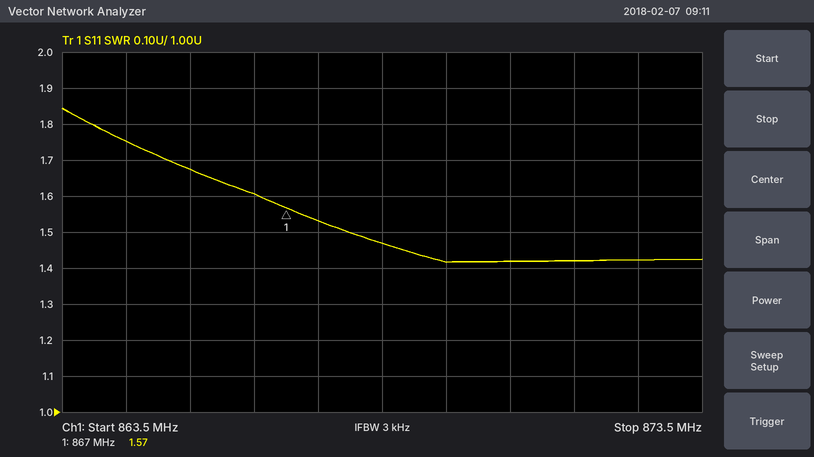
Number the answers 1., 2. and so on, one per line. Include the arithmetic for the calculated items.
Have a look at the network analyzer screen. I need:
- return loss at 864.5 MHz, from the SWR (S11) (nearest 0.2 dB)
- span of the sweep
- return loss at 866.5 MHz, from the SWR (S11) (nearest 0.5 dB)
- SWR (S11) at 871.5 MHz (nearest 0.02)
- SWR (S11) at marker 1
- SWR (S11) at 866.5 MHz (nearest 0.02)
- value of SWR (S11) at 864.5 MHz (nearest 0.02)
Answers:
1. −20 log10((1.76 − 1)/(1.76 + 1)) ≈ 11.2 dB
2. 10 MHz
3. −20 log10((1.6 − 1)/(1.6 + 1)) ≈ 12.7 dB, so 12.5 dB to the nearest 0.5 dB
4. 1.42
5. 1.57
6. 1.60
7. 1.76
